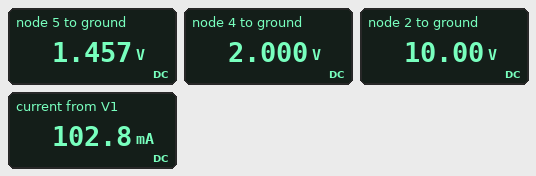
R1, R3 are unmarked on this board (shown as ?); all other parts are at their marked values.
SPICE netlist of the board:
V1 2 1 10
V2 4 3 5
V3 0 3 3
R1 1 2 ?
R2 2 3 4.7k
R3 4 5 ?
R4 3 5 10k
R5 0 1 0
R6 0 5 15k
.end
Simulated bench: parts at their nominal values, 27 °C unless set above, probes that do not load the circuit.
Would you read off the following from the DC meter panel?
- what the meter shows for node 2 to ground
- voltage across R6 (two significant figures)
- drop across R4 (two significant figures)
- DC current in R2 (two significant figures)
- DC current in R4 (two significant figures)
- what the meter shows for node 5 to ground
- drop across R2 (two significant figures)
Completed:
10.00 V
1.5 V
4.5 V
2.8 mA
450 µA
1.457 V
13 V
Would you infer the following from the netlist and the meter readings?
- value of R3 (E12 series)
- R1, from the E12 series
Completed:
1 kΩ
100 Ω
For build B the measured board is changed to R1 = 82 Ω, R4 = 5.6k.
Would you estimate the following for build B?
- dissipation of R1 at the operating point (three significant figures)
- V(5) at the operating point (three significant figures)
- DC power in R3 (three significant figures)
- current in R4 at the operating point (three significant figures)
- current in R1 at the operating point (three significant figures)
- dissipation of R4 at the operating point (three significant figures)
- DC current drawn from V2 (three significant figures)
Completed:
1.22 W
1.18 V
679 µW
746 µA
122 mA
3.11 mW
824 µA
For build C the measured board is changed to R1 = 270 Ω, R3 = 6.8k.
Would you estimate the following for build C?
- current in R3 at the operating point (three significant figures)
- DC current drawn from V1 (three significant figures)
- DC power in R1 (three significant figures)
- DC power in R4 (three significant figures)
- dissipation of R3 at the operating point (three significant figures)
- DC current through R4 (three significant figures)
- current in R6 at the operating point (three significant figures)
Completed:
297 µA
39.8 mA
370 mW
889 µW
599 µW
298 µA
1.25 µA
